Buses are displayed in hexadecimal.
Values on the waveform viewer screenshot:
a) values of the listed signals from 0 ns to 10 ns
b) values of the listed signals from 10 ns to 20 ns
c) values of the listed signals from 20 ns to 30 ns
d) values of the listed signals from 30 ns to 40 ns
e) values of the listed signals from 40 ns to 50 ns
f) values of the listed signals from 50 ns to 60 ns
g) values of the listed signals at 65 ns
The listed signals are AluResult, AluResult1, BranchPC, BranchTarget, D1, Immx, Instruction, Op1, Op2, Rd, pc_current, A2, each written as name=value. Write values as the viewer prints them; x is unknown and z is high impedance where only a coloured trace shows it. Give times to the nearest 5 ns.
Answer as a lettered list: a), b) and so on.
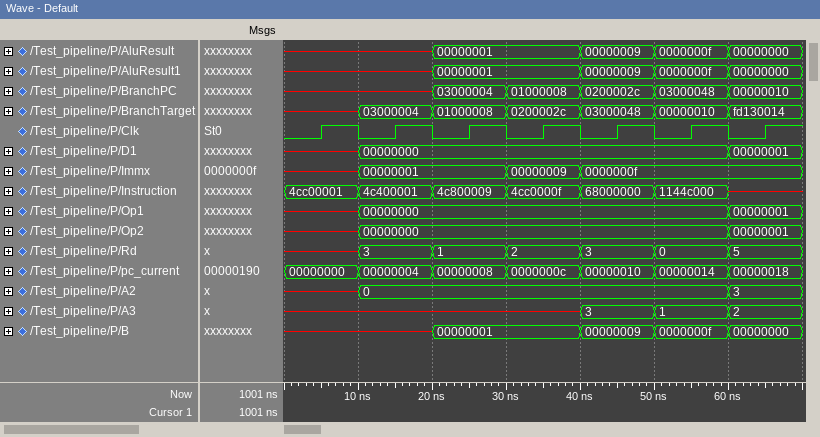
a) AluResult=x, AluResult1=x, BranchPC=x, BranchTarget=x, D1=x, Immx=x, Instruction=4cc00001, Op1=x, Op2=x, Rd=x, pc_current=00000000, A2=x
b) AluResult=x, AluResult1=x, BranchPC=x, BranchTarget=03000004, D1=00000000, Immx=00000001, Instruction=4c400001, Op1=00000000, Op2=00000000, Rd=3, pc_current=00000004, A2=0
c) AluResult=00000001, AluResult1=00000001, BranchPC=03000004, BranchTarget=01000008, D1=00000000, Immx=00000001, Instruction=4c800009, Op1=00000000, Op2=00000000, Rd=1, pc_current=00000008, A2=0
d) AluResult=00000001, AluResult1=00000001, BranchPC=01000008, BranchTarget=0200002c, D1=00000000, Immx=00000009, Instruction=4cc0000f, Op1=00000000, Op2=00000000, Rd=2, pc_current=0000000c, A2=0
e) AluResult=00000009, AluResult1=00000009, BranchPC=0200002c, BranchTarget=03000048, D1=00000000, Immx=0000000f, Instruction=68000000, Op1=00000000, Op2=00000000, Rd=3, pc_current=00000010, A2=0
f) AluResult=0000000f, AluResult1=0000000f, BranchPC=03000048, BranchTarget=00000010, D1=00000000, Immx=0000000f, Instruction=1144c000, Op1=00000000, Op2=00000000, Rd=0, pc_current=00000014, A2=0
g) AluResult=00000000, AluResult1=00000000, BranchPC=00000010, BranchTarget=fd130014, D1=00000001, Immx=0000000f, Instruction=x, Op1=00000001, Op2=00000001, Rd=5, pc_current=00000018, A2=3
